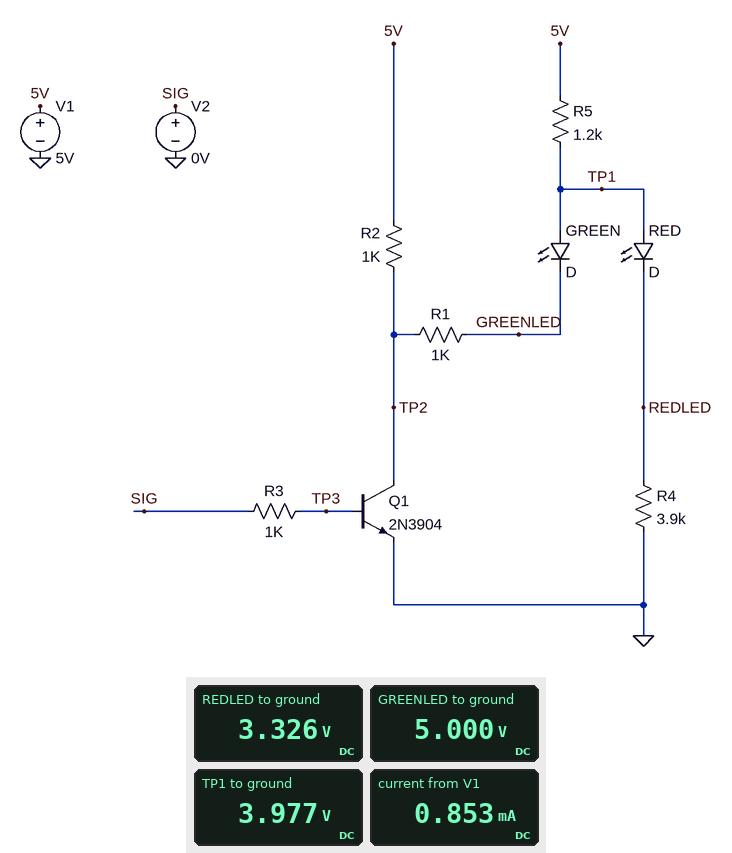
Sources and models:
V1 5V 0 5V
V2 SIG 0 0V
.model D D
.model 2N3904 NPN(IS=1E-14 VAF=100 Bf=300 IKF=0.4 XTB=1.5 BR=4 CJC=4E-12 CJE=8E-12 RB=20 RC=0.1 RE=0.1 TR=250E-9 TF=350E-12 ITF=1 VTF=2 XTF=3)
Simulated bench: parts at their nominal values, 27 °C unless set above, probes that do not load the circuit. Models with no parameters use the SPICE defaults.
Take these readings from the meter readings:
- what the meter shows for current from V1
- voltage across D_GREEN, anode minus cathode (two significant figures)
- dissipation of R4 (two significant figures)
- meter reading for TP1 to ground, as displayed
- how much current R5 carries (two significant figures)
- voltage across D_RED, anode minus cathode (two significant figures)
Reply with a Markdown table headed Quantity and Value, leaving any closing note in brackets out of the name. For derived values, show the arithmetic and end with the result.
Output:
| Quantity | Value |
|---|---|
| what the meter shows for current from V1 | 0.853 mA |
| voltage across D_GREEN, anode minus cathode | 3.977 V - 5 V = -1.0 V |
| dissipation of R4 | (3.326 V)^2 / 3.9 kΩ = 2.8 mW |
| meter reading for TP1 to ground, as displayed | 3.977 V |
| how much current R5 carries | (5 V - 3.977 V) / 1.2 kΩ = 850 µA |
| voltage across D_RED, anode minus cathode | 3.977 V - 3.326 V = 650 mV |
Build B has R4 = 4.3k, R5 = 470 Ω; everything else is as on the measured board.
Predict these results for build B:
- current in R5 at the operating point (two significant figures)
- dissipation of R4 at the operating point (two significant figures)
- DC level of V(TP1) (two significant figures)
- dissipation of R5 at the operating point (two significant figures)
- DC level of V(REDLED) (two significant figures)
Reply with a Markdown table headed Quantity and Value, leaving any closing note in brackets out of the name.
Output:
| Quantity | Value |
|---|---|
| current in R5 at the operating point | 910 µA |
| dissipation of R4 at the operating point | 3.6 mW |
| DC level of V(TP1) | 4.6 V |
| dissipation of R5 at the operating point | 390 µW |
| DC level of V(REDLED) | 3.9 V |
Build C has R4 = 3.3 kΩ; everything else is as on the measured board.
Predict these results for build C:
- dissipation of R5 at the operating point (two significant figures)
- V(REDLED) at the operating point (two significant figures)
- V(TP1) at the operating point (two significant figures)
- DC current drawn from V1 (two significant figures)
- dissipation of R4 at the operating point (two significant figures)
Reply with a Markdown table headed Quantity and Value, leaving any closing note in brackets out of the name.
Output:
| Quantity | Value |
|---|---|
| dissipation of R5 at the operating point | 1.1 mW |
| V(REDLED) at the operating point | 3.2 V |
| V(TP1) at the operating point | 3.8 V |
| DC current drawn from V1 | 970 µA |
| dissipation of R4 at the operating point | 3.1 mW |
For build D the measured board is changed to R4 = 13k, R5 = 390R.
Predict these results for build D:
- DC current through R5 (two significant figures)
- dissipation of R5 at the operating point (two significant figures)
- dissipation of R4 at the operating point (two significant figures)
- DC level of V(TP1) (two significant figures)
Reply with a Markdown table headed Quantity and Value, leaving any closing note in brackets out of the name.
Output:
| Quantity | Value |
|---|---|
| DC current through R5 | 330 µA |
| dissipation of R5 at the operating point | 42 µW |
| dissipation of R4 at the operating point | 1.4 mW |
| DC level of V(TP1) | 4.9 V |
